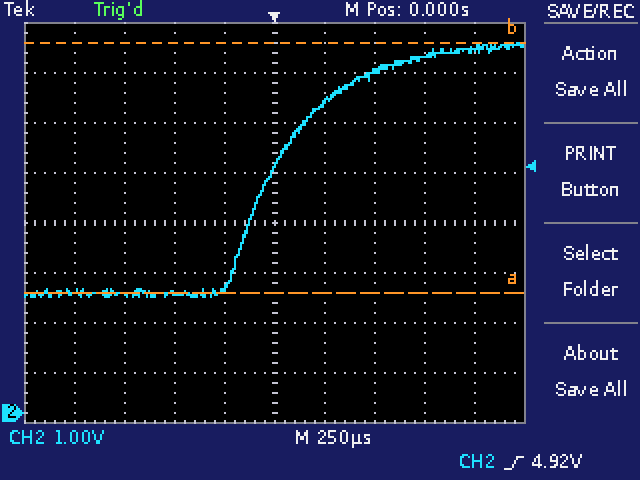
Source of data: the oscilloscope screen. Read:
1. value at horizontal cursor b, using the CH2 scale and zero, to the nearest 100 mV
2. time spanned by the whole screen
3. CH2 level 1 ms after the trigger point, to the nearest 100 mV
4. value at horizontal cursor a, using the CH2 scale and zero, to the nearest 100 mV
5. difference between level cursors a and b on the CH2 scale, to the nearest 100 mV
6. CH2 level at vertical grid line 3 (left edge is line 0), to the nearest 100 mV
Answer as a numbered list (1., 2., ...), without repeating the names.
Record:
1. 7.4 V
2. 2.5 ms
3. 7.3 V
4. 2.4 V
5. 5.0 V
6. 2.4 V
